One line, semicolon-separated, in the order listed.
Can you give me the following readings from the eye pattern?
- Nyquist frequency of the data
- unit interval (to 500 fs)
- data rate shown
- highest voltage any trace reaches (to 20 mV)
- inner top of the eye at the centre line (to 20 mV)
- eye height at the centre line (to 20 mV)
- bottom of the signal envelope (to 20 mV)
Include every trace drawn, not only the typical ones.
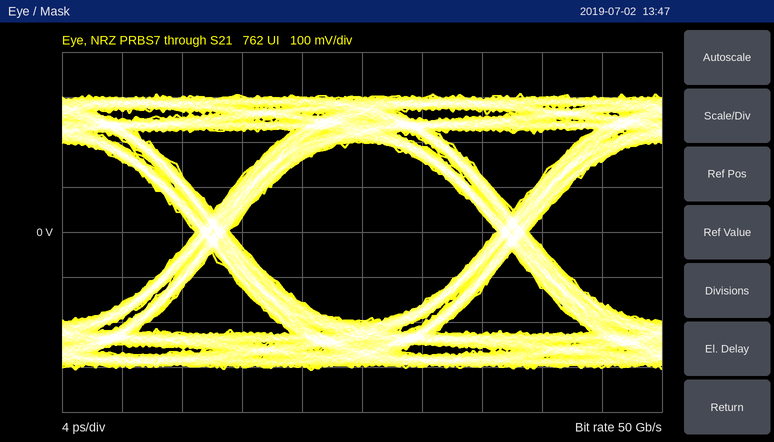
25 GHz; 20.0 ps; 50 Gb/s; 300 mV; 200 mV; 400 mV; -300 mV
